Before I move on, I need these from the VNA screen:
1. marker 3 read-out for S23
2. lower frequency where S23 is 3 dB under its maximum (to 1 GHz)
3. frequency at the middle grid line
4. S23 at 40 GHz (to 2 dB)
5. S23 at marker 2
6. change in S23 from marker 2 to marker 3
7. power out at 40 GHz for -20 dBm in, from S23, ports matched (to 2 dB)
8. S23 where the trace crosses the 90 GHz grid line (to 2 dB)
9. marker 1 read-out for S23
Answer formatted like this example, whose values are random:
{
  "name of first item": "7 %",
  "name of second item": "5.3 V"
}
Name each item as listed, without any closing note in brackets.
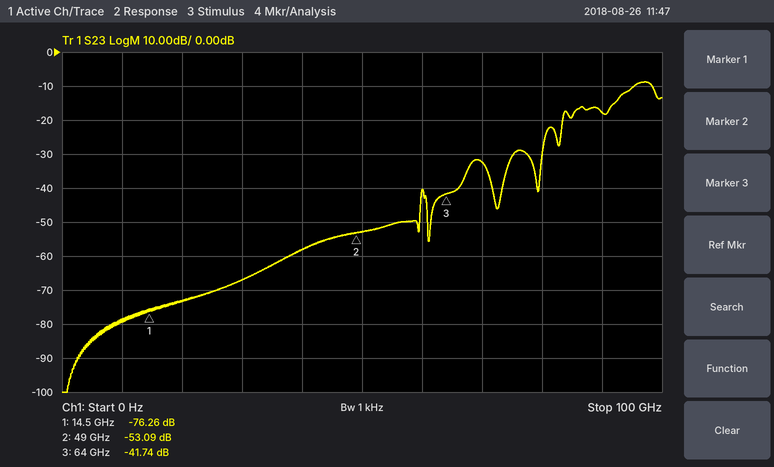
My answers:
{
  "marker 3 read-out for S23": "-41.74 dB",
  "lower frequency where S23 is 3 dB under its maximum": "94 GHz",
  "frequency at the middle grid line": "50 GHz",
  "S23 at 40 GHz": "-58 dB",
  "S23 at marker 2": "-53.09 dB",
  "change in S23 from marker 2 to marker 3": "11.35 dB",
  "power out at 40 GHz for -20 dBm in, from S23, ports matched": "-78 dBm",
  "S23 where the trace crosses the 90 GHz grid line": "-18 dB",
  "marker 1 read-out for S23": "-76.26 dB"
}
